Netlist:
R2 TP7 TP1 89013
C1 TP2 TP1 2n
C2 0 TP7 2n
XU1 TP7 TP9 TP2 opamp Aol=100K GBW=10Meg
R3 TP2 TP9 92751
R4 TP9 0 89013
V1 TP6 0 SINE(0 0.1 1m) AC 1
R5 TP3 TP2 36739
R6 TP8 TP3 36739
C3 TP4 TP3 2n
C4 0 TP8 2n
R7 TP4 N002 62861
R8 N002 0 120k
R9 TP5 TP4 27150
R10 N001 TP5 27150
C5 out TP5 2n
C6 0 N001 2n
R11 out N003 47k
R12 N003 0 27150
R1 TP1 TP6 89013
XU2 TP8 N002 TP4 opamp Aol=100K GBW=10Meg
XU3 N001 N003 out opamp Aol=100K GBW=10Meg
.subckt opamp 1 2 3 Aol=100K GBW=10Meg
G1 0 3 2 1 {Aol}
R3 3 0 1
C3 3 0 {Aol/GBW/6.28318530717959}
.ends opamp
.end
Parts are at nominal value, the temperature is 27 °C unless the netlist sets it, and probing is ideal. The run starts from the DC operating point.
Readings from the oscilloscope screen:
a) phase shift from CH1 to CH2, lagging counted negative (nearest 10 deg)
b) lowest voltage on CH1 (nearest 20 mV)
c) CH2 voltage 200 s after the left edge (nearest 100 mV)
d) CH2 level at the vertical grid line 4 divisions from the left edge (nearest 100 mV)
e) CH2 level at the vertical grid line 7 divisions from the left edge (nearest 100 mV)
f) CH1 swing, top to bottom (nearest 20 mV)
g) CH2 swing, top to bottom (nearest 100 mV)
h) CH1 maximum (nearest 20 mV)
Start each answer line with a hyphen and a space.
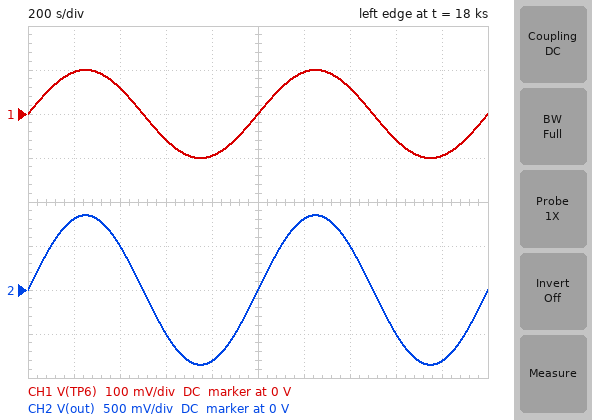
- 0 deg
- -100 mV
- 800 mV
- -800 mV
- 500 mV
- 200 mV
- 1.7 V
- 100 mV
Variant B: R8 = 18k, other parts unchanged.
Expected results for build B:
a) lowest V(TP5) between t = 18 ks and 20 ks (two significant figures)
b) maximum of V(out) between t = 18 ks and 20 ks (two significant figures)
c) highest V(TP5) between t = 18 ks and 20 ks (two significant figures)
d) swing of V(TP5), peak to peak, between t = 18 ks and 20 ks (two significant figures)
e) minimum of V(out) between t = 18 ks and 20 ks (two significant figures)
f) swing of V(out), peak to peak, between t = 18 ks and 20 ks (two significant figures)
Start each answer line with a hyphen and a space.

- -920 mV
- 2.5 V
- 920 mV
- 1.8 V
- -2.5 V
- 5.0 V
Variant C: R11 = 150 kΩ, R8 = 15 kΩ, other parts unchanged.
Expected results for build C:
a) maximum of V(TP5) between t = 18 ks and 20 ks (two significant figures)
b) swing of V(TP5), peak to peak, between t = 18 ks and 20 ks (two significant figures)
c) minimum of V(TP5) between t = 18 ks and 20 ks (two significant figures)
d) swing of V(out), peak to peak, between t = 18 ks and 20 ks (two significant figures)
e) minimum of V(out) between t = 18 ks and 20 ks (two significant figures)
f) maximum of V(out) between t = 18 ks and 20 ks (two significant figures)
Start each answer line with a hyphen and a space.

- 1.1 V
- 2.1 V
- -1.1 V
- 14 V
- -6.9 V
- 6.9 V
